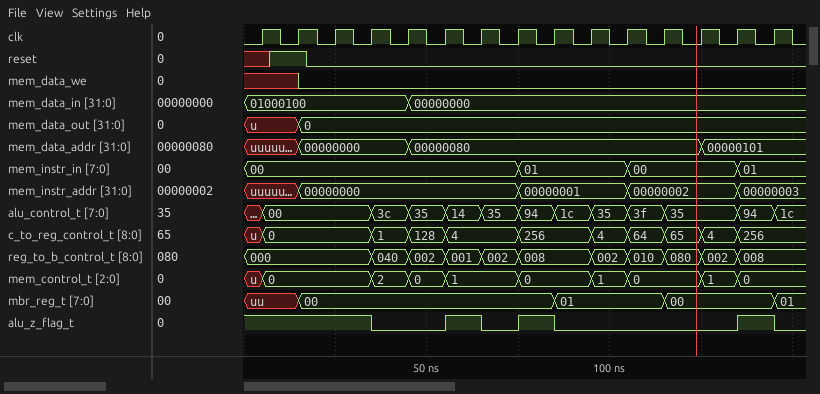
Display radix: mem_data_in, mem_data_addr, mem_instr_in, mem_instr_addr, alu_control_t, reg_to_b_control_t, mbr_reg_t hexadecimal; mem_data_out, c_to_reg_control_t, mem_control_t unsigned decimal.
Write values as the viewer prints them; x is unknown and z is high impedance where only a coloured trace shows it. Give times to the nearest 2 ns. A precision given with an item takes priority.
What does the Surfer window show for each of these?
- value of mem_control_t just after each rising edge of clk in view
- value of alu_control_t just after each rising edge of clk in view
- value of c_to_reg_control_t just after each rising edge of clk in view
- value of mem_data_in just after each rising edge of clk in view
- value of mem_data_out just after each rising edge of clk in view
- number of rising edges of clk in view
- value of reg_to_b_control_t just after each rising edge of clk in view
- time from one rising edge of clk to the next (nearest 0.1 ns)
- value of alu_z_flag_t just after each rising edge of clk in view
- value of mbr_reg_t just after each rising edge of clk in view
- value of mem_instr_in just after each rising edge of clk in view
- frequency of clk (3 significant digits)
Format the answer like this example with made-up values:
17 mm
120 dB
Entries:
0, 0, 0, 2, 0, 1, 1, 0, 0, 1, 0, 0, 1, 0, 0
00, 00, 00, 3c, 35, 14, 35, 94, 1c, 35, 3f, 35, 35, 94, 1c
0, 0, 0, 1, 128, 4, 4, 256, 256, 4, 64, 65, 4, 256, 256
01000100, 01000100, 01000100, 01000100, 00000000, 00000000, 00000000, 00000000, 00000000, 00000000, 00000000, 00000000, 00000000, 00000000, 00000000
u, 0, 0, 0, 0, 0, 0, 0, 0, 0, 0, 0, 0, 0, 0
15
000, 000, 000, 040, 002, 001, 002, 008, 008, 002, 010, 080, 002, 008, 008
10 ns
1 1 1 0 0 1 0 1 0 0 0 0 0 1 0
uu, 00, 00, 00, 00, 00, 00, 00, 01, 01, 01, 00, 00, 00, 01
00, 00, 00, 00, 00, 00, 00, 01, 01, 01, 00, 00, 00, 01, 01
100 MHz
